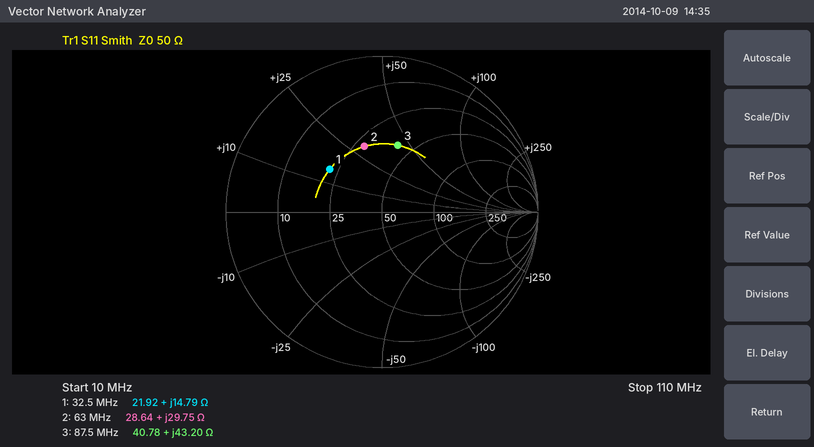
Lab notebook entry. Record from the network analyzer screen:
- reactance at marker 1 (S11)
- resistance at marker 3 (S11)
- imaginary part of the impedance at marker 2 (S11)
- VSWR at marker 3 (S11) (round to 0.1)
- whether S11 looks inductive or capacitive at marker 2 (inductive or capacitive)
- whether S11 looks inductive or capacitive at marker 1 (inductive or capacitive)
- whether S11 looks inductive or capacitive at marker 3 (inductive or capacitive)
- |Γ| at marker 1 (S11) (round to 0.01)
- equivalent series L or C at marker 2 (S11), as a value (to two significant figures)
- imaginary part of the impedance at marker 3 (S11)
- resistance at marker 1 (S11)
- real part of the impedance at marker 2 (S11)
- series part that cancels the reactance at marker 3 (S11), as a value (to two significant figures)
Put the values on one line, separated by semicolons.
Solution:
+14.79 Ω; 40.78 Ω; +29.75 Ω; 2.6; inductive; inductive; inductive; 0.43; 75 nH; +43.20 Ω; 21.92 Ω; 28.64 Ω; 42 pF
